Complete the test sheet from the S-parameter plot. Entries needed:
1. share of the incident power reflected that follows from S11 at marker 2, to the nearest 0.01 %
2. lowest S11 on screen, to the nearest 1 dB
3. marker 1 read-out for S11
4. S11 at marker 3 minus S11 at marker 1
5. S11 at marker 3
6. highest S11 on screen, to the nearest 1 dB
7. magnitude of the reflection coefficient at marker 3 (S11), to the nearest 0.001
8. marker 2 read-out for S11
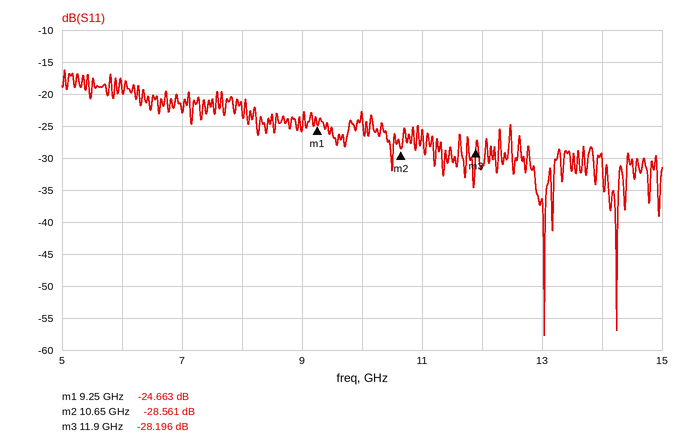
0.14 %
-58 dB
-24.663 dB
-3.533 dB
-28.196 dB
-16 dB
0.039
-28.561 dB
